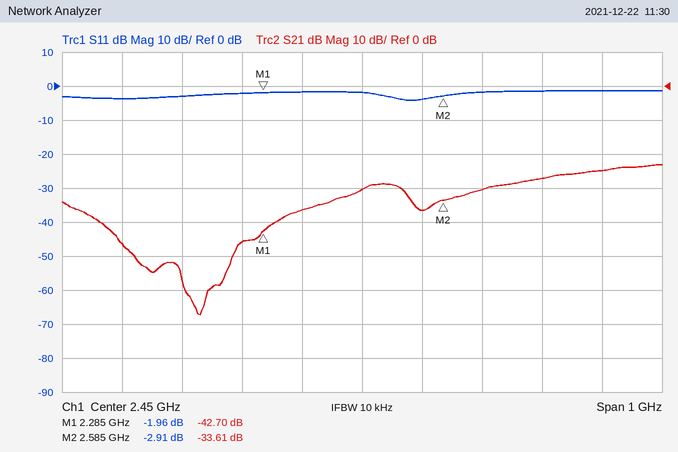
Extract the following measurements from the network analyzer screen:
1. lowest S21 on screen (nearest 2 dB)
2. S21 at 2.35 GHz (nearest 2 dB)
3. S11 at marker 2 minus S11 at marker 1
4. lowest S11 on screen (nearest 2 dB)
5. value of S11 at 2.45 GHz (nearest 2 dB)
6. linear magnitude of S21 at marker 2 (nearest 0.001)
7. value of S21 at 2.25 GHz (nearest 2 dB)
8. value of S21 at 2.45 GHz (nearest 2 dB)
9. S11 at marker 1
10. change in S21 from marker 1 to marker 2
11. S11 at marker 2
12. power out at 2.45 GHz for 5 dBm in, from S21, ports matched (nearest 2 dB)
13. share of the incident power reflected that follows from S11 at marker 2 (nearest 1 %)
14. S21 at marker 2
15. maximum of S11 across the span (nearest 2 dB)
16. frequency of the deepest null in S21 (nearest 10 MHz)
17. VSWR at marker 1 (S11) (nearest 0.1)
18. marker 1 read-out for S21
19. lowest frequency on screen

-68 dB
-36 dB
-0.95 dB
-4 dB
-2 dB
0.021
-46 dB
-30 dB
-1.96 dB
9.09 dB
-2.91 dB
-26 dBm
51 %
-33.61 dB
-2 dB
2.18 GHz
8.9
-42.70 dB
1.95 GHz
